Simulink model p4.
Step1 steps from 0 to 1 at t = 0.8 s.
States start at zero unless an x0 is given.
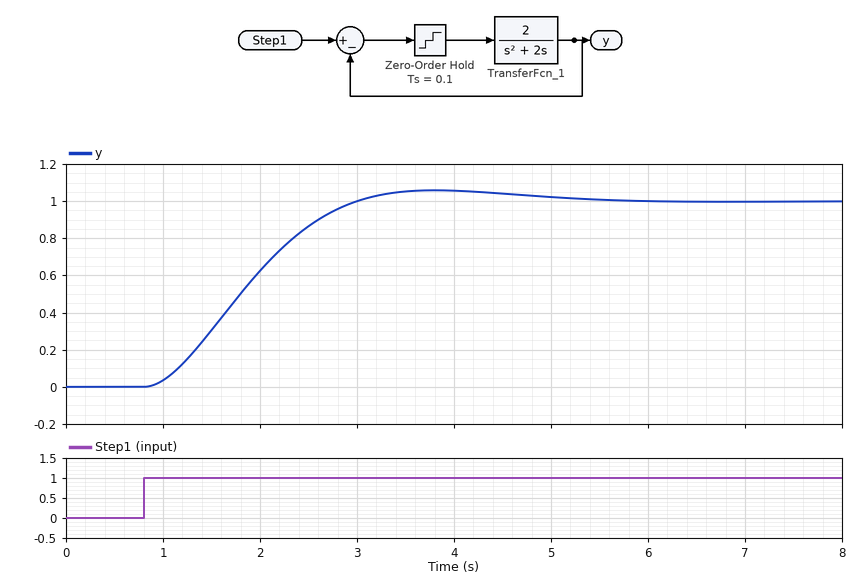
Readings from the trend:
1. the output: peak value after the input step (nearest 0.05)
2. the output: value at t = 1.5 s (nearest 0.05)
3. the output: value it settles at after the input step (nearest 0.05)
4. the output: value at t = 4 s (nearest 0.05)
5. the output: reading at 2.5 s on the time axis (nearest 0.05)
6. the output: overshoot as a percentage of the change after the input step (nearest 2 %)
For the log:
1.05
0.30
1.00
1.05
0.85
6 %
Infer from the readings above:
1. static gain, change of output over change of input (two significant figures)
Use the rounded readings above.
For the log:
1.0
